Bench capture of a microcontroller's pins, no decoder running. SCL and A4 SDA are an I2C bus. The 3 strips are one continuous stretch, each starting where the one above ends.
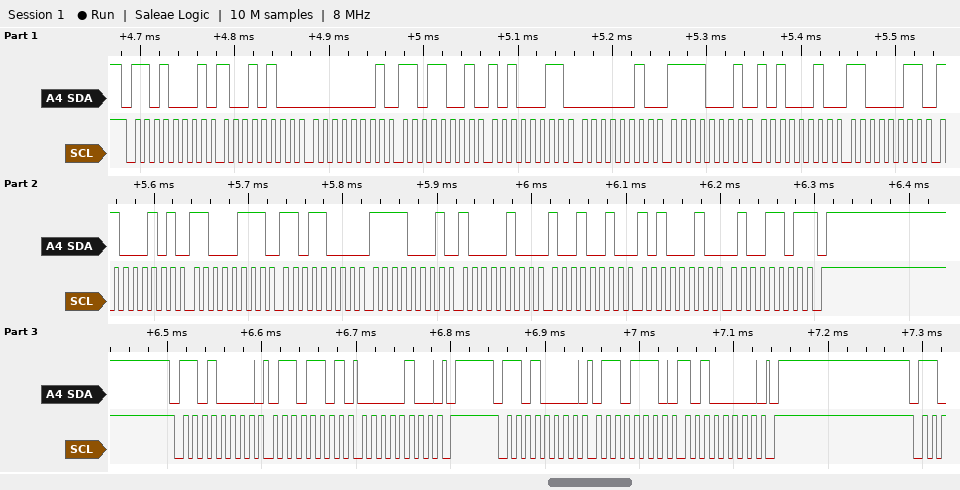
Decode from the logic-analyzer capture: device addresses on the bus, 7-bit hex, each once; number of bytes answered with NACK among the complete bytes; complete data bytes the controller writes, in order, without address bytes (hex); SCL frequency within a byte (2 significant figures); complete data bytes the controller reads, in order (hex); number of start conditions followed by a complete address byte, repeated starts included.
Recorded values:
0x68
1
6D 04 6E A0
100 kHz
94 01 D9 A3 02 F1 A2 C3 C5 C7 D8 F1 84 92 A2 4D
3
